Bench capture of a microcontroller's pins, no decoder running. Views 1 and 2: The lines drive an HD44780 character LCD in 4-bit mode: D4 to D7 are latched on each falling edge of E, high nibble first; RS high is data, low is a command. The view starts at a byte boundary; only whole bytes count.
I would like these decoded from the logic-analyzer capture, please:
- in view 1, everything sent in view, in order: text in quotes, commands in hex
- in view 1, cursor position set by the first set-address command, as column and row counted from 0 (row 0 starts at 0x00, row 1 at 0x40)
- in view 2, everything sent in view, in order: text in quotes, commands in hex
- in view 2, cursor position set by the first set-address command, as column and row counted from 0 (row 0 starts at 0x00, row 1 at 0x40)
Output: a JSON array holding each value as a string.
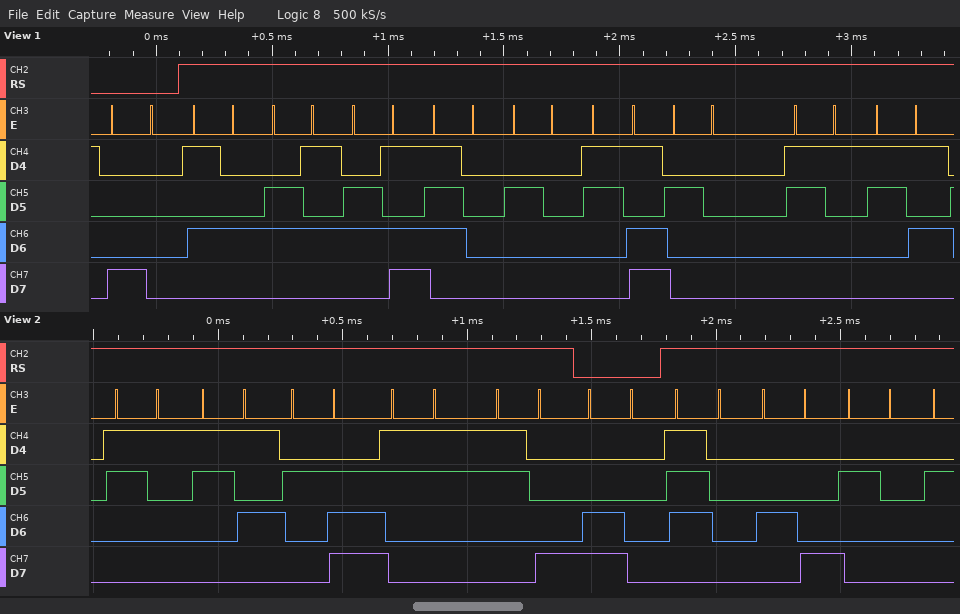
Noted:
["0x80 \"Temp = 15\"", "column 0, row 0", "\"15.38\" 0xC0 \"pH \"", "column 0, row 1"]
